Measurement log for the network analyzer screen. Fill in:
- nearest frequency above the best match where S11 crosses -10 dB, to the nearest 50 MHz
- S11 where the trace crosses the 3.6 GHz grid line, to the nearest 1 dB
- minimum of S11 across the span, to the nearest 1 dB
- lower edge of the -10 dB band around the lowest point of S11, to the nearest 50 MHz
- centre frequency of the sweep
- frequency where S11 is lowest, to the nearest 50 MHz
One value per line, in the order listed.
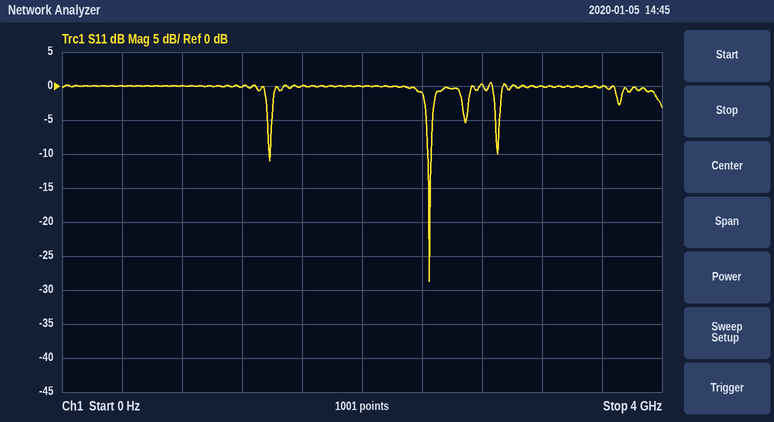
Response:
2.45 GHz
0 dB
-29 dB
2.45 GHz
2 GHz
2.45 GHz
